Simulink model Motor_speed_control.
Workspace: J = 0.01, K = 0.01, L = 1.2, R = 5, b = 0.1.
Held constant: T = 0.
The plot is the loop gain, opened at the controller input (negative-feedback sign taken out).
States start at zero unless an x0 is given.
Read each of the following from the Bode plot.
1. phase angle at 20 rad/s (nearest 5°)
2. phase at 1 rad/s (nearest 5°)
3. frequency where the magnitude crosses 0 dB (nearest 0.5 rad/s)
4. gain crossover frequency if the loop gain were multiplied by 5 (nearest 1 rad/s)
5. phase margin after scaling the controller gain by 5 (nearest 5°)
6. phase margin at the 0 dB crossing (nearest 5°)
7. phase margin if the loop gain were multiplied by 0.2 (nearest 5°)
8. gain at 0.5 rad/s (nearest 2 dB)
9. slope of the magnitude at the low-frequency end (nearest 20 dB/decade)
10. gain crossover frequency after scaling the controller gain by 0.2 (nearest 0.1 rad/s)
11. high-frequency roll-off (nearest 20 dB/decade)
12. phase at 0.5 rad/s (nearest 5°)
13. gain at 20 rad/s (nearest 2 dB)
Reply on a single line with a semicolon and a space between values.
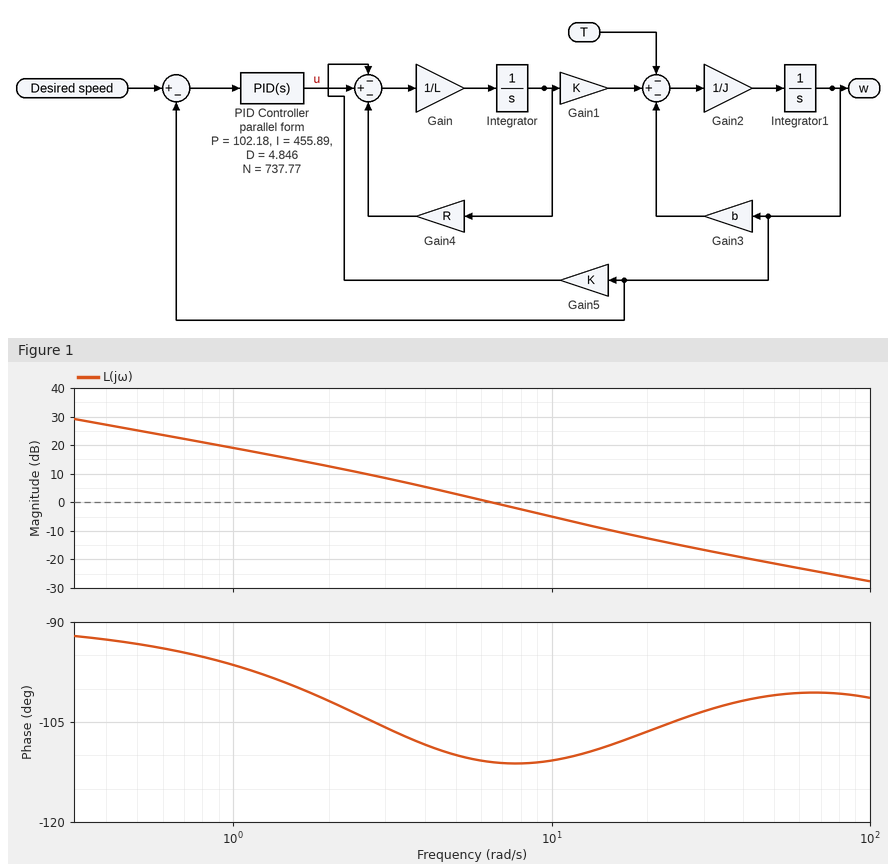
-105°; -95°; 6.5 rad/s; 23 rad/s; 75°; 70°; 80°; 26 dB; -20 dB/decade; 1.7 rad/s; -20 dB/decade; -95°; -12 dB
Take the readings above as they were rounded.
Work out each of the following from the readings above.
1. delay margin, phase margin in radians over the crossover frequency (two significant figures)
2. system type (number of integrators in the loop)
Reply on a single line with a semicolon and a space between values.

0.19 s; 1
